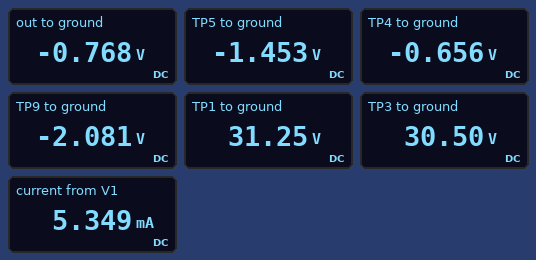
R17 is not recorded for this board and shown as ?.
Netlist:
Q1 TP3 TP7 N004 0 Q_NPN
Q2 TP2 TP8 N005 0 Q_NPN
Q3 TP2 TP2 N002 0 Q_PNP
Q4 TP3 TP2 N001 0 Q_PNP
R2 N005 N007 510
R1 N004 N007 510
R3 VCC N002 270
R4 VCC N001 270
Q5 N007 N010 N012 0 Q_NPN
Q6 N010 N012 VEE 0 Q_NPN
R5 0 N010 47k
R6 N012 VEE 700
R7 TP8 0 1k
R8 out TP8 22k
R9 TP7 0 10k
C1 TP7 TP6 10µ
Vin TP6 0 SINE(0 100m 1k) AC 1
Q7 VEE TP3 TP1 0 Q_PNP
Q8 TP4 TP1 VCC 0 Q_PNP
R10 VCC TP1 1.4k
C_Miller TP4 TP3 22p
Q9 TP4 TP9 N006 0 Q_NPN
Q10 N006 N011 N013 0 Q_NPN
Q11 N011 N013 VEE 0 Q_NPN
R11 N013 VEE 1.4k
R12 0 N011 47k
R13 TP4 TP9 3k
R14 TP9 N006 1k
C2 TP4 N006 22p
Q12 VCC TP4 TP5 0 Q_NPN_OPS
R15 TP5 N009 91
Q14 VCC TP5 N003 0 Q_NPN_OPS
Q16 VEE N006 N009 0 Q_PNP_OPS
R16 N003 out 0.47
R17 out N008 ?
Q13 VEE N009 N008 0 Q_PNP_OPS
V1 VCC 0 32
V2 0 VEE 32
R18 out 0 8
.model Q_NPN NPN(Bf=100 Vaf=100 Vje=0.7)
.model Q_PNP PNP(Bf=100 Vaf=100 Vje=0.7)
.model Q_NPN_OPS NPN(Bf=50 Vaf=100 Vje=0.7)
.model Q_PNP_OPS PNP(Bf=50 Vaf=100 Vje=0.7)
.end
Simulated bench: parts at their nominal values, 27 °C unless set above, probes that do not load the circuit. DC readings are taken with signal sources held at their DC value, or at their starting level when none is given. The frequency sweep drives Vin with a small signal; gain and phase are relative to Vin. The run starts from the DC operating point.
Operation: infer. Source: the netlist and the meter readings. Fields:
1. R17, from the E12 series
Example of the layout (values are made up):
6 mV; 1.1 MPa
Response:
1 Ω
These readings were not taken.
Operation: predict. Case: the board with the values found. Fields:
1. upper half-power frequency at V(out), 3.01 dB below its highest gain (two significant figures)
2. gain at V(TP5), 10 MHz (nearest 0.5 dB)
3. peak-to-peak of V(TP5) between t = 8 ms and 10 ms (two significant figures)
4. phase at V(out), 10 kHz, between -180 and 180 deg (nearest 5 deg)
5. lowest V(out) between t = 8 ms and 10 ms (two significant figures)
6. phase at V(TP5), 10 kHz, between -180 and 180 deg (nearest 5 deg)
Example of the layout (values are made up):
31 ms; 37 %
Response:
440 kHz; 2.0 dB; 6.8 V; 0 deg; -3.1 V; 0 deg
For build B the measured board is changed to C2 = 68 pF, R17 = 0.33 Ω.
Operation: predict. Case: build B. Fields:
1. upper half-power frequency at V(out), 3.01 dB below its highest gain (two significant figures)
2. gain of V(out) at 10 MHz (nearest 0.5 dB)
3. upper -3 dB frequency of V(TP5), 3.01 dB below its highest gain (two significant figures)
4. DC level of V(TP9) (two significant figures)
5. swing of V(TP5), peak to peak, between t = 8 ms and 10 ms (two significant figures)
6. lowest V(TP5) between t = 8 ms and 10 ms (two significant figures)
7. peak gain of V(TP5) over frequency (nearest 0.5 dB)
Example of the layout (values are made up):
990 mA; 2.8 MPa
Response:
470 kHz; 1.5 dB; 460 kHz; -2.0 V; 6.5 V; -4.0 V; 28.5 dB
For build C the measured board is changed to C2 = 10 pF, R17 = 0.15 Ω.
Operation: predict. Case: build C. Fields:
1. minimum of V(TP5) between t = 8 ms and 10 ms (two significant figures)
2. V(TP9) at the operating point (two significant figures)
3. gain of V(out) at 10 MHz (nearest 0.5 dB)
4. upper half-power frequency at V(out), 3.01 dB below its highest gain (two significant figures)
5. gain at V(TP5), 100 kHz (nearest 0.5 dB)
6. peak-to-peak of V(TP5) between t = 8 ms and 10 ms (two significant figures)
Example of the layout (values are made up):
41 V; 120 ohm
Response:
-3.9 V; -2.0 V; 1.5 dB; 490 kHz; 28.0 dB; 6.4 V
